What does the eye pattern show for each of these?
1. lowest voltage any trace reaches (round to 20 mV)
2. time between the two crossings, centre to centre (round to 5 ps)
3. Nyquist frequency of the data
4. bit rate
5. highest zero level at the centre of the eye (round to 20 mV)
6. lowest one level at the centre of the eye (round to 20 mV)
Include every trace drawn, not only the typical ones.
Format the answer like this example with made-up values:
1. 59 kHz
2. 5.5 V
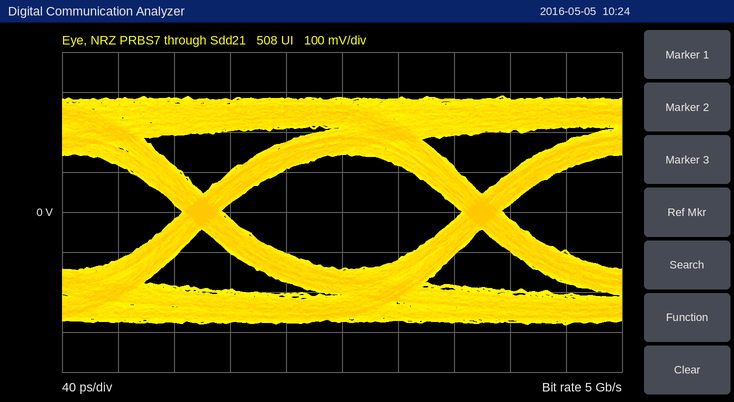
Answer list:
1. -280 mV
2. 200 ps
3. 2.5 GHz
4. 5 Gb/s
5. -140 mV
6. 140 mV
